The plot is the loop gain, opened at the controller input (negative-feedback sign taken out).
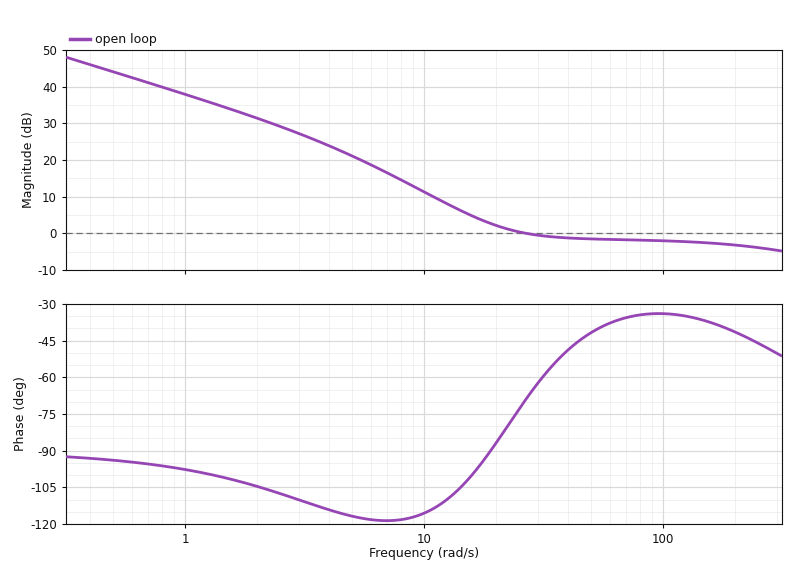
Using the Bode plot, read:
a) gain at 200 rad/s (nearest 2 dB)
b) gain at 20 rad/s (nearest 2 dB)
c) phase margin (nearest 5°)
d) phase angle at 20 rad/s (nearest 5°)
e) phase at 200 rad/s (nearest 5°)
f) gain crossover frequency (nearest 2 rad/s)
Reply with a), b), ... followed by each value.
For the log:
a) -4 dB
b) 2 dB
c) 110°
d) -85°
e) -40°
f) 26 rad/s
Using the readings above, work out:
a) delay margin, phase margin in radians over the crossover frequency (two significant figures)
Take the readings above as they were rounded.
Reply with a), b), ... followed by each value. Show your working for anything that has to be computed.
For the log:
a) 110 × π / 180 / 26 = 0.074 s
